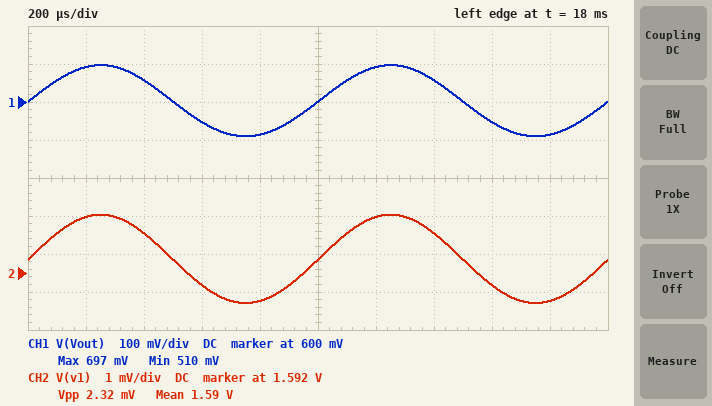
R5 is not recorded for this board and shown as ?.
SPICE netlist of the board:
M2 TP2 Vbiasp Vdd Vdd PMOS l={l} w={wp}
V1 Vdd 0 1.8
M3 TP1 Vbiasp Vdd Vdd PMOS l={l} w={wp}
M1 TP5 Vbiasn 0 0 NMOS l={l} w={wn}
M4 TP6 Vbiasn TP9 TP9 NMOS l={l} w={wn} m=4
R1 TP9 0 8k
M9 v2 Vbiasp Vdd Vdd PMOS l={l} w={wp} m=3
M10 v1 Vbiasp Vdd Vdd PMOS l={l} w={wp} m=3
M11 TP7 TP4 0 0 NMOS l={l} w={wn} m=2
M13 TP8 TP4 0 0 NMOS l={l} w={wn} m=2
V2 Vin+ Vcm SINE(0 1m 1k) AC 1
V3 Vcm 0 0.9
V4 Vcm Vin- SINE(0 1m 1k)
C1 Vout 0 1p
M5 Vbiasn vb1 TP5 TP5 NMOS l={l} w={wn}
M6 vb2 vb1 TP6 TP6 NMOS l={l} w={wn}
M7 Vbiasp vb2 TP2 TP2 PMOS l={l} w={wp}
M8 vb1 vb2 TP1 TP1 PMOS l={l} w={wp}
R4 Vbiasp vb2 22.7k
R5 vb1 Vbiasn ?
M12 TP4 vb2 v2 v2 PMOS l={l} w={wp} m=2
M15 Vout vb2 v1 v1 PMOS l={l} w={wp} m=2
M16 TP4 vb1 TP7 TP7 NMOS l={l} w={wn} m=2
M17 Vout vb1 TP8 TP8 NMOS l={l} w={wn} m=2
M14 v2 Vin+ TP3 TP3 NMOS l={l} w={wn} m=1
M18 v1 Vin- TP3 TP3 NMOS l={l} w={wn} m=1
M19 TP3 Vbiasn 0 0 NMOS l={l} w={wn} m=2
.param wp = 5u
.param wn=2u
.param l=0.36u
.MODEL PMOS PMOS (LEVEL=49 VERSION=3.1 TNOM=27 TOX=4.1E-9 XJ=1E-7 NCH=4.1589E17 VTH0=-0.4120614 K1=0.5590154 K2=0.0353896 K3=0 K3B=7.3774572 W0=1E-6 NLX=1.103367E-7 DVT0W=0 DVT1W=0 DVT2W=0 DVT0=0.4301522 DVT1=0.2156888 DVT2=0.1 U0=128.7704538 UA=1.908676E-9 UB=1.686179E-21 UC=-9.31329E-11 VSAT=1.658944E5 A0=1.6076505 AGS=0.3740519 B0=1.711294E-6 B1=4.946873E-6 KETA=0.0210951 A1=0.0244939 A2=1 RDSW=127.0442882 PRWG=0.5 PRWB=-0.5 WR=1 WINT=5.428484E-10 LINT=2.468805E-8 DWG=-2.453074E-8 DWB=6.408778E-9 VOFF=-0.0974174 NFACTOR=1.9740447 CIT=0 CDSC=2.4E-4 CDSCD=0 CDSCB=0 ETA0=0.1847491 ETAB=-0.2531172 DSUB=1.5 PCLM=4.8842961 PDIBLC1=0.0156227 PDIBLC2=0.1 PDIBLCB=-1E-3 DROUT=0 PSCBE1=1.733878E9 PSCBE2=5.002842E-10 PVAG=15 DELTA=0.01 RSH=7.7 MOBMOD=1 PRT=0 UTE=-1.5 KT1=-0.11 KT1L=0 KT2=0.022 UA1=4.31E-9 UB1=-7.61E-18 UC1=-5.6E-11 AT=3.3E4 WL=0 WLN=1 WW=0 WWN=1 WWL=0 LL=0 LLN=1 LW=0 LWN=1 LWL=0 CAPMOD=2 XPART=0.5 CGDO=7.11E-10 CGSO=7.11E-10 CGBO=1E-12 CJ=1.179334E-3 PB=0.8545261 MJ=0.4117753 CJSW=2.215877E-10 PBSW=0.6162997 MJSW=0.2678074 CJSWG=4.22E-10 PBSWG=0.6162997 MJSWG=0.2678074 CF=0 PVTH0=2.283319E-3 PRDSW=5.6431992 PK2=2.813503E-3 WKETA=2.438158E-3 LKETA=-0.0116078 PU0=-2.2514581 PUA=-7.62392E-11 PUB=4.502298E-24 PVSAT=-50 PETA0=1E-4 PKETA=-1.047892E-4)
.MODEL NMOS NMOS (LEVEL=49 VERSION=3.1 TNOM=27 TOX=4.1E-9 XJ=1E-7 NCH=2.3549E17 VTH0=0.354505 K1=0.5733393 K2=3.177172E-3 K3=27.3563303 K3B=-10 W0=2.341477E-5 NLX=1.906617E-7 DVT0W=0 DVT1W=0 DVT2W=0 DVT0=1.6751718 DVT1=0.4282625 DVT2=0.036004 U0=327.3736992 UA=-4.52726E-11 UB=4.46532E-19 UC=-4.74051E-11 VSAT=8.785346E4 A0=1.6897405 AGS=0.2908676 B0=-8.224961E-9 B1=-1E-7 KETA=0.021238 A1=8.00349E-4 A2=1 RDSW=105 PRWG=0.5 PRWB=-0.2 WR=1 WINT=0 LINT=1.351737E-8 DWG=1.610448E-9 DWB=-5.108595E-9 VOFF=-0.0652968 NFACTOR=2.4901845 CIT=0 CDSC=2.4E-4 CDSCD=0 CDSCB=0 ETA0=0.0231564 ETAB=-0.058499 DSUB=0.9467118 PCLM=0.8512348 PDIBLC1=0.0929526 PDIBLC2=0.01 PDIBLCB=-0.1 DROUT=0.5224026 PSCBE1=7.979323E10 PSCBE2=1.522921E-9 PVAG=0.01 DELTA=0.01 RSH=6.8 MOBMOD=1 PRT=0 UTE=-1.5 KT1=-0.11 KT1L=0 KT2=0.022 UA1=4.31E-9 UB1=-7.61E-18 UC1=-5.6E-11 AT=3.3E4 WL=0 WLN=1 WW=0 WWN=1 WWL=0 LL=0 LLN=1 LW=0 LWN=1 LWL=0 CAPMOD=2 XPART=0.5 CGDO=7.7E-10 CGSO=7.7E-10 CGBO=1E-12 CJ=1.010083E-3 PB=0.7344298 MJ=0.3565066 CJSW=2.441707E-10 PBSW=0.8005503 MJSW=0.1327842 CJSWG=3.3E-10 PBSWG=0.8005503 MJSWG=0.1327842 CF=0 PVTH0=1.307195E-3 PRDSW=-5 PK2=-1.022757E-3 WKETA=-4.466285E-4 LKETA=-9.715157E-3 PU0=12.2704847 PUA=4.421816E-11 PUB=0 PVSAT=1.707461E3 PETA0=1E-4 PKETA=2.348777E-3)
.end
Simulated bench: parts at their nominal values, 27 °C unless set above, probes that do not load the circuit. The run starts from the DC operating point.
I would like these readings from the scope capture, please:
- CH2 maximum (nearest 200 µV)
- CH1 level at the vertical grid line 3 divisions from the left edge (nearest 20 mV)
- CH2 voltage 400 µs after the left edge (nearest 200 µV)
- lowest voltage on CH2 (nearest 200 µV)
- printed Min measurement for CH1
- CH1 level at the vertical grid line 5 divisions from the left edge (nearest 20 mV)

1.5936 V
540 mV
1.5930 V
1.5912 V
510 mV
600 mV
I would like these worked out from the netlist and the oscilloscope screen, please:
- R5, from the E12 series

120 kΩ
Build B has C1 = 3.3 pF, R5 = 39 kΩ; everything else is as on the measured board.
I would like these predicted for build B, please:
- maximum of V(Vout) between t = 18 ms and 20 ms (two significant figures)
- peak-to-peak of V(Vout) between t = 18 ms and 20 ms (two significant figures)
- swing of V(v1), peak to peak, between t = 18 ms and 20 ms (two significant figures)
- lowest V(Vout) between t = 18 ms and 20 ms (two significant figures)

1.5 V
1.2 V
29 mV
320 mV
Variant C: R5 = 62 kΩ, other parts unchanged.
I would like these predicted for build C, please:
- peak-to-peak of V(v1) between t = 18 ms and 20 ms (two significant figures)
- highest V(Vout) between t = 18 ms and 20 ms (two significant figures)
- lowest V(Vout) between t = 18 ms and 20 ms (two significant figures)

23 mV
1.5 V
470 mV
